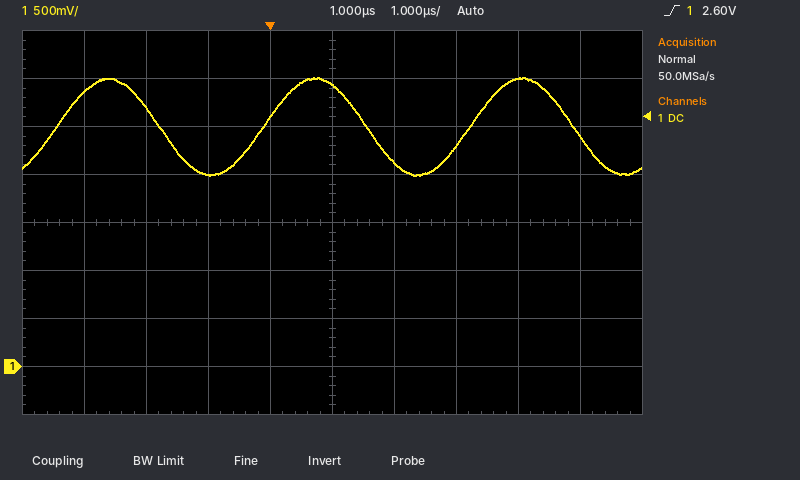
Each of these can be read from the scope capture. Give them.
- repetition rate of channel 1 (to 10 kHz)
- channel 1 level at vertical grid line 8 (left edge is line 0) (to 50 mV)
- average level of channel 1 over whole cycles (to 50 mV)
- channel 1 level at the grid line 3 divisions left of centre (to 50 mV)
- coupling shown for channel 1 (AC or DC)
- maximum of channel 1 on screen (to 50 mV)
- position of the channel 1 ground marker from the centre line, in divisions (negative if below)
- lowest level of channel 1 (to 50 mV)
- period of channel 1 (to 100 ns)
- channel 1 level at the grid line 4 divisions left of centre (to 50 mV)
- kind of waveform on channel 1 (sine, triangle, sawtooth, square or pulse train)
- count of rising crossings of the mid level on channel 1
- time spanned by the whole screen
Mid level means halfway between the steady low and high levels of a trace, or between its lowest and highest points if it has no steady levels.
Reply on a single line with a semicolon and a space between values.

300 kHz; 3.00 V; 2.50 V; 2.70 V; DC; 3.00 V; -3.0 div; 2.00 V; 3.3 µs; 2.85 V; sine; 3; 10 µs
